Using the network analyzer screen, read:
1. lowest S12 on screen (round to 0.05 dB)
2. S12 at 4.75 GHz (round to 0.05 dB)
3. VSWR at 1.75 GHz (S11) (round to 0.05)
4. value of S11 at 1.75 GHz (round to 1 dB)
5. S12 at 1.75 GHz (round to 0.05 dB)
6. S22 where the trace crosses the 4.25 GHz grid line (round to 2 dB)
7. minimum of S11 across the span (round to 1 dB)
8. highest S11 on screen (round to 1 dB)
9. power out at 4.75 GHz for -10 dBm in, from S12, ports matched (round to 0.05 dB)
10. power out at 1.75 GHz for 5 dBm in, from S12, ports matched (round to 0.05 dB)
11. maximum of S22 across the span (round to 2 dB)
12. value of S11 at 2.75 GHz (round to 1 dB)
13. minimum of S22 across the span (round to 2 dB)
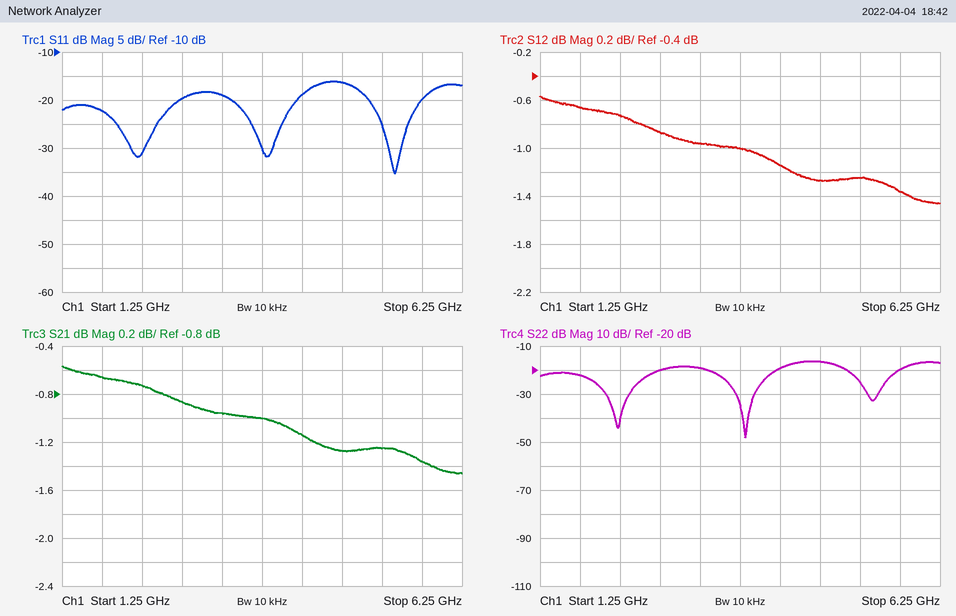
-1.45 dB
-1.25 dB
1.15
-22 dB
-0.65 dB
-20 dB
-35 dB
-16 dB
-11.25 dBm
4.35 dBm
-16 dB
-20 dB
-48 dB
